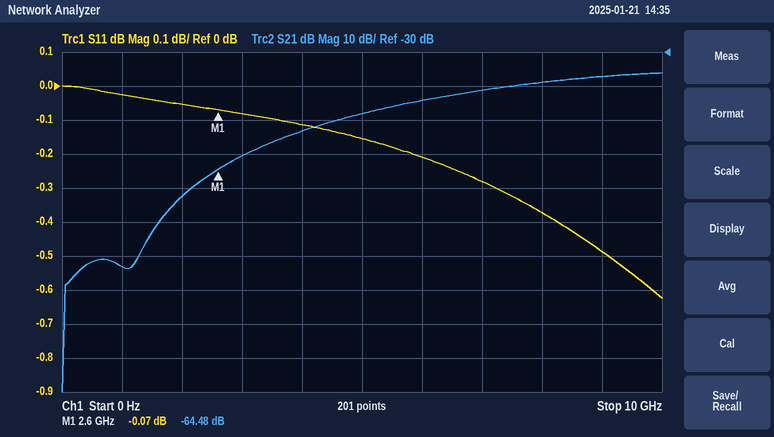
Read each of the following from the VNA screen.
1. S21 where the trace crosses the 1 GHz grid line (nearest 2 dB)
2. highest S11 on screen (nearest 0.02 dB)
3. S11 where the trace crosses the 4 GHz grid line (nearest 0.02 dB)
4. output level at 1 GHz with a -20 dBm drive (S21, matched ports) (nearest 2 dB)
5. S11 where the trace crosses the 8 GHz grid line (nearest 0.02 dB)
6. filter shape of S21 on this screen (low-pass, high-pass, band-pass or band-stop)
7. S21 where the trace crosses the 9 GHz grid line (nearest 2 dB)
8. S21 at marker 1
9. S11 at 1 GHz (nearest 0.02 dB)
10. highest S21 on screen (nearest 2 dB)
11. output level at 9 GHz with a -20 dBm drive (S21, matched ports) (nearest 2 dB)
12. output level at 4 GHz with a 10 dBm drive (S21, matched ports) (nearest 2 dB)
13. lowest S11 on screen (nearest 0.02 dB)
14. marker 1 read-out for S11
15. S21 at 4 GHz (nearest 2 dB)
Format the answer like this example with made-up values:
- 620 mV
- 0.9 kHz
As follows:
- -94 dB
- 0.00 dB
- -0.12 dB
- -114 dBm
- -0.38 dB
- high-pass
- -38 dB
- -64.48 dB
- -0.02 dB
- -36 dB
- -58 dBm
- -44 dBm
- -0.62 dB
- -0.07 dB
- -54 dB
